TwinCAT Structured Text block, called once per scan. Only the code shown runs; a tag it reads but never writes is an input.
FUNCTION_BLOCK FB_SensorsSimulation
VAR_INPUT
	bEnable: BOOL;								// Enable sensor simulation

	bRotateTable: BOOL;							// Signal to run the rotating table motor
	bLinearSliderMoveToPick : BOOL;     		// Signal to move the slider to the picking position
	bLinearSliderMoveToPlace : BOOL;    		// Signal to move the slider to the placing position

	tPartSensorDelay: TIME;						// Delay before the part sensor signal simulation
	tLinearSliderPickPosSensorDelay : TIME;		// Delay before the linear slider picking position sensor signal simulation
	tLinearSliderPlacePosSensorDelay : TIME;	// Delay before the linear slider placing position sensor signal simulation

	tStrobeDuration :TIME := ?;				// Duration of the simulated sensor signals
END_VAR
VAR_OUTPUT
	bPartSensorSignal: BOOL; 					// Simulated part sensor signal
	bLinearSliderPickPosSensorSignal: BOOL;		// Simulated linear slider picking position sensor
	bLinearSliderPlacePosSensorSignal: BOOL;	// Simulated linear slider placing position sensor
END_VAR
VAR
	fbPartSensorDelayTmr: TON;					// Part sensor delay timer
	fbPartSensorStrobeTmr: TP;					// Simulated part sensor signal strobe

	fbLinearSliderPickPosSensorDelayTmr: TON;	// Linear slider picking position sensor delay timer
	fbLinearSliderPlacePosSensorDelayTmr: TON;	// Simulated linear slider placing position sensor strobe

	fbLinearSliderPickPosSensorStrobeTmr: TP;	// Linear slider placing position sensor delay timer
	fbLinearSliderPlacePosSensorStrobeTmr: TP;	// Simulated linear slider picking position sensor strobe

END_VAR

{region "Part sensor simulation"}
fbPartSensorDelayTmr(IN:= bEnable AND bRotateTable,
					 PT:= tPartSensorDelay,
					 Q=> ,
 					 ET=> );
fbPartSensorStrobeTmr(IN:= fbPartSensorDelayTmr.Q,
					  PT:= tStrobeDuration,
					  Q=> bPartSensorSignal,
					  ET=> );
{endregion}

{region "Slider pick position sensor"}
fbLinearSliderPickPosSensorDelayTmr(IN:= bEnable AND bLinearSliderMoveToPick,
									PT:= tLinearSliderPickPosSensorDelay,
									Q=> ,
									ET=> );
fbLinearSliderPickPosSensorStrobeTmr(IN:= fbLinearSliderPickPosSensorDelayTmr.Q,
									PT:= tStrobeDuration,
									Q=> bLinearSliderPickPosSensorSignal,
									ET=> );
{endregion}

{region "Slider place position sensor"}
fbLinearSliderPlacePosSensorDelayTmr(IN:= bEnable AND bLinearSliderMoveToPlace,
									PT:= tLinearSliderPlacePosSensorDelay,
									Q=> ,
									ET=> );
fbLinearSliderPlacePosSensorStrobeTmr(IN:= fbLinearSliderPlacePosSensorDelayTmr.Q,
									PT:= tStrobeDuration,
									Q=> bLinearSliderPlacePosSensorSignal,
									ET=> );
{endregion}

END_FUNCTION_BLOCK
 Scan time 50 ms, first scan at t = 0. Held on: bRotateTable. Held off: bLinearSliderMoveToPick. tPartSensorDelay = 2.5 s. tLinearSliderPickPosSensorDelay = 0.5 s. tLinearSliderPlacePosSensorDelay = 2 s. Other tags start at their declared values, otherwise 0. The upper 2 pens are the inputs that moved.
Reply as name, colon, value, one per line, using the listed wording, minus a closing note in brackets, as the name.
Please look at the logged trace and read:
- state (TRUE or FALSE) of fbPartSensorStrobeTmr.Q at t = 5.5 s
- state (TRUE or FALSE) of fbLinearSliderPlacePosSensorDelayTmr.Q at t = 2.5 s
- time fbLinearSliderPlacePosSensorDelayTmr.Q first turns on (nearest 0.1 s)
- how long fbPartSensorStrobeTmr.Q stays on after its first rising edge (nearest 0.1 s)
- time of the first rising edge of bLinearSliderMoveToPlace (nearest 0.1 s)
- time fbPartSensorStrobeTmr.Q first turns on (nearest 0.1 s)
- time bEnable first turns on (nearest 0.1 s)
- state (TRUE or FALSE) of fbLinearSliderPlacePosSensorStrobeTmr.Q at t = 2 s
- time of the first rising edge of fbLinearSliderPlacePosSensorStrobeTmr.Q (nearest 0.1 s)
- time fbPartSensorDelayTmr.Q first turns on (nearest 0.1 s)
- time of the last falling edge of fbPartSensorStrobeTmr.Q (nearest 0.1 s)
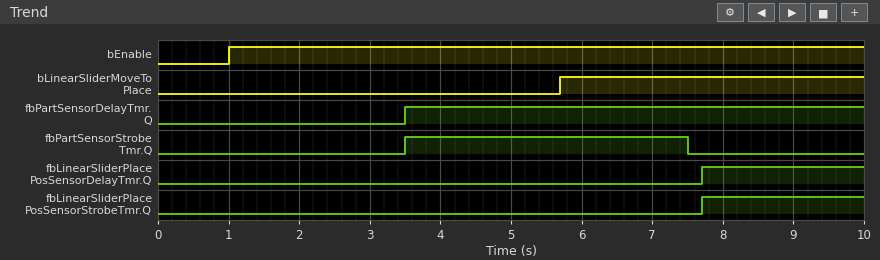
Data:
state (TRUE or FALSE) of fbPartSensorStrobeTmr.Q at t = 5.5 s: TRUE
state (TRUE or FALSE) of fbLinearSliderPlacePosSensorDelayTmr.Q at t = 2.5 s: FALSE
time fbLinearSliderPlacePosSensorDelayTmr.Q first turns on: 7.7 s
how long fbPartSensorStrobeTmr.Q stays on after its first rising edge: 4.0 s
time of the first rising edge of bLinearSliderMoveToPlace: 5.7 s
time fbPartSensorStrobeTmr.Q first turns on: 3.5 s
time bEnable first turns on: 1.0 s
state (TRUE or FALSE) of fbLinearSliderPlacePosSensorStrobeTmr.Q at t = 2 s: FALSE
time of the first rising edge of fbLinearSliderPlacePosSensorStrobeTmr.Q: 7.7 s
time fbPartSensorDelayTmr.Q first turns on: 3.5 s
time of the last falling edge of fbPartSensorStrobeTmr.Q: 7.5 s
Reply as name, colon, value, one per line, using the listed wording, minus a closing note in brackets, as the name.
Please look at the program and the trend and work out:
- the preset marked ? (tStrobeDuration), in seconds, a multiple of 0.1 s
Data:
the preset marked ? (tStrobeDuration), in seconds, a multiple of 0.1 s: 4.0 s
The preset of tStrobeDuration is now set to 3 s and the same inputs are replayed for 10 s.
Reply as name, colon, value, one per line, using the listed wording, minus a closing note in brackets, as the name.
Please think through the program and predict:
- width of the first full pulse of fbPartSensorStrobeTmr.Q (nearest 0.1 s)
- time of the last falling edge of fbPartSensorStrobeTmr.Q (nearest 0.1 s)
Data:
width of the first full pulse of fbPartSensorStrobeTmr.Q: 3.0 s
time of the last falling edge of fbPartSensorStrobeTmr.Q: 6.5 s
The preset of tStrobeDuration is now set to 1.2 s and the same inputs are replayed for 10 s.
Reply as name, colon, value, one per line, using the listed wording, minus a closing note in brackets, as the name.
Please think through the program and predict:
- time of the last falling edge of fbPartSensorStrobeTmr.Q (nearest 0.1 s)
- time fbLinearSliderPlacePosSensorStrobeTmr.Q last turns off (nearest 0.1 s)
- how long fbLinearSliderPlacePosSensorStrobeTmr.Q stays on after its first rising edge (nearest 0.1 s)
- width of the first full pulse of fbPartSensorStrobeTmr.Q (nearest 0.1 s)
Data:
time of the last falling edge of fbPartSensorStrobeTmr.Q: 4.7 s
time fbLinearSliderPlacePosSensorStrobeTmr.Q last turns off: 8.9 s
how long fbLinearSliderPlacePosSensorStrobeTmr.Q stays on after its first rising edge: 1.2 s
width of the first full pulse of fbPartSensorStrobeTmr.Q: 1.2 s
